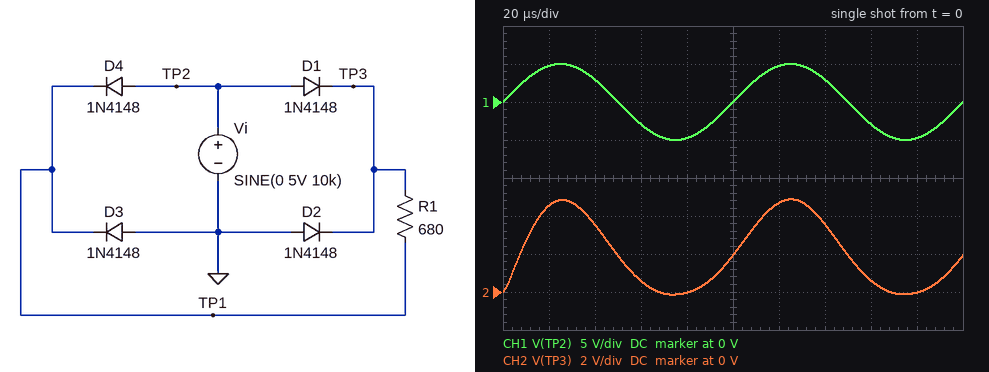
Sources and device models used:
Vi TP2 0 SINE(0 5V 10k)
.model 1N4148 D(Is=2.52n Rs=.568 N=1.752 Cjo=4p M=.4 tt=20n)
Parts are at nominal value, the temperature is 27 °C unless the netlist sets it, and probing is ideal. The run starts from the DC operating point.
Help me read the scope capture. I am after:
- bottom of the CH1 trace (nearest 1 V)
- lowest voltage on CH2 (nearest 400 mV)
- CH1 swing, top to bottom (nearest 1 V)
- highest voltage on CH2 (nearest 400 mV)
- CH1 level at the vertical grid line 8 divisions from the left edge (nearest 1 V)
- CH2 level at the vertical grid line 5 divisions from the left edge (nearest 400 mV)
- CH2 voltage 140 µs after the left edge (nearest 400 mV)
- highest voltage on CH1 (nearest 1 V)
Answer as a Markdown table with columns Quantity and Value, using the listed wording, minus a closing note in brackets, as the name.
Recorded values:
| Quantity | Value |
|---|---|
| bottom of the CH1 trace | -5 V |
| lowest voltage on CH2 | 0 V |
| CH1 swing, top to bottom | 10 V |
| highest voltage on CH2 | 4.8 V |
| CH1 level at the vertical grid line 8 divisions from the left edge | -3 V |
| CH2 level at the vertical grid line 5 divisions from the left edge | 2.0 V |
| CH2 voltage 140 µs after the left edge | 3.6 V |
| highest voltage on CH1 | 5 V |
